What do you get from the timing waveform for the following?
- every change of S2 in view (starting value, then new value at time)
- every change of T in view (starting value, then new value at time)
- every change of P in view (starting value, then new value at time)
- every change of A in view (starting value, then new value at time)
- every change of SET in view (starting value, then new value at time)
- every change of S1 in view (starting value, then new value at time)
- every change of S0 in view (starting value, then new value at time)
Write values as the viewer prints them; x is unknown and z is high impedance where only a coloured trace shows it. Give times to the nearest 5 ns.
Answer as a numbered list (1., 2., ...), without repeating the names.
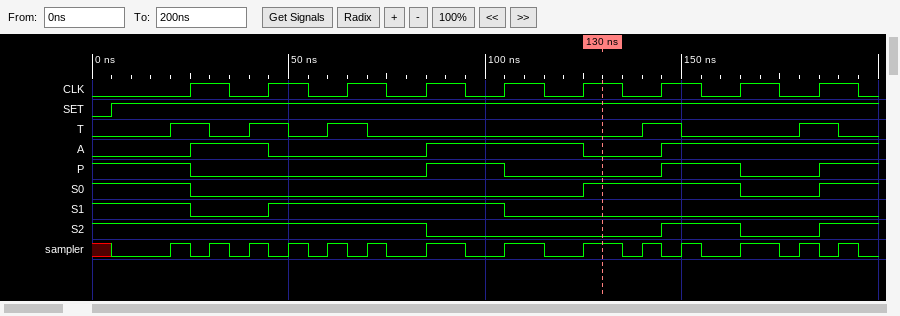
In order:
1. 1, 0 at 85 ns, 1 at 145 ns, 0 at 165 ns, 1 at 185 ns
2. 0, 1 at 20 ns, 0 at 30 ns, 1 at 40 ns, 0 at 50 ns, 1 at 60 ns, 0 at 70 ns, 1 at 140 ns, 0 at 150 ns, 1 at 180 ns, 0 at 190 ns
3. 1, 0 at 25 ns, 1 at 85 ns, 0 at 105 ns, 1 at 145 ns, 0 at 165 ns, 1 at 185 ns
4. 0, 1 at 25 ns, 0 at 45 ns, 1 at 85 ns, 0 at 125 ns, 1 at 145 ns
5. 0, 1 at 5 ns
6. 1, 0 at 25 ns, 1 at 45 ns, 0 at 105 ns
7. 1, 0 at 25 ns, 1 at 125 ns, 0 at 165 ns, 1 at 185 ns
